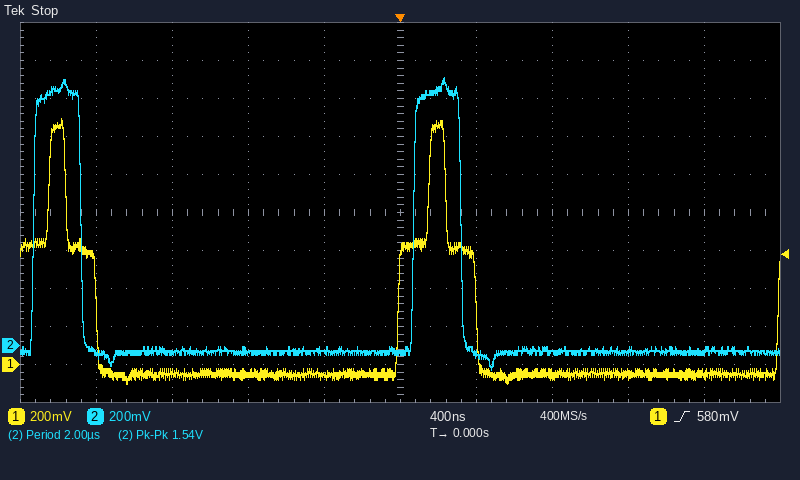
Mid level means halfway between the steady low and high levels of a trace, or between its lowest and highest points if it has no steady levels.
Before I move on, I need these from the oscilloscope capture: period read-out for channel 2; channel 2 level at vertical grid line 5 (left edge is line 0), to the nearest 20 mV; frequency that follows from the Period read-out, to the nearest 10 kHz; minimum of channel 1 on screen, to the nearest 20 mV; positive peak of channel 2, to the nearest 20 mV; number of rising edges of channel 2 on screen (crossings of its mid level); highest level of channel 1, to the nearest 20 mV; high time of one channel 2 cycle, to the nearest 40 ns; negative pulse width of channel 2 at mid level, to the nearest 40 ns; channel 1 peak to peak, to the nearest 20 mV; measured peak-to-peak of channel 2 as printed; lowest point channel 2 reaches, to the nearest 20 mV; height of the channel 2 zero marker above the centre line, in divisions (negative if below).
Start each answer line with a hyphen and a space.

- 2.00 µs
- -40 mV
- 500 kHz
- -100 mV
- 1.42 V
- 2
- 1.30 V
- 240 ns
- 1.76 µs
- 1.40 V
- 1.54 V
- -120 mV
- -3.5 div
